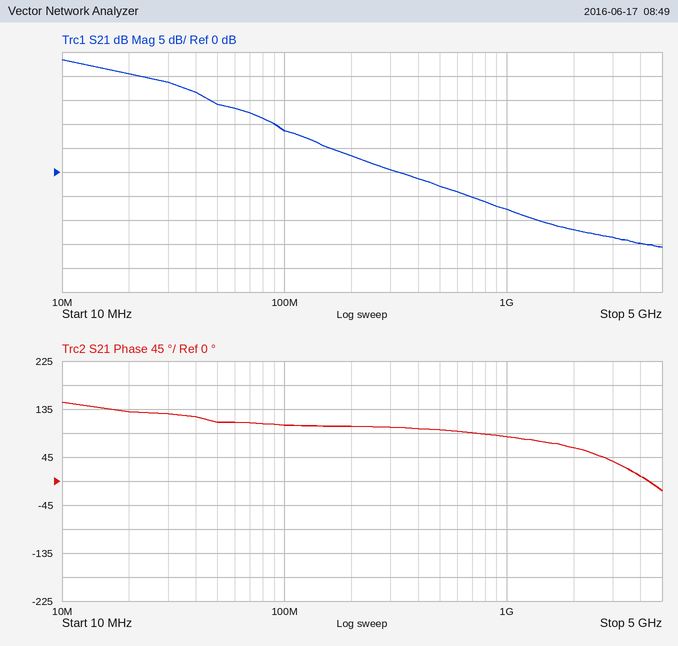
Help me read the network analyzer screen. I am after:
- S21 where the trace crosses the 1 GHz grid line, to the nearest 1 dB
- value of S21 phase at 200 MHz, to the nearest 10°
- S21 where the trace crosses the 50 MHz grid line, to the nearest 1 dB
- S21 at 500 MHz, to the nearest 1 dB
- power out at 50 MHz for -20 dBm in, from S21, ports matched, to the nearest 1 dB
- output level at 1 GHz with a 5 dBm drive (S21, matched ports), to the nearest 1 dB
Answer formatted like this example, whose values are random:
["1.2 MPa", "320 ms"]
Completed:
["-8 dB", "100°", "14 dB", "-3 dB", "-6 dBm", "-3 dBm"]
